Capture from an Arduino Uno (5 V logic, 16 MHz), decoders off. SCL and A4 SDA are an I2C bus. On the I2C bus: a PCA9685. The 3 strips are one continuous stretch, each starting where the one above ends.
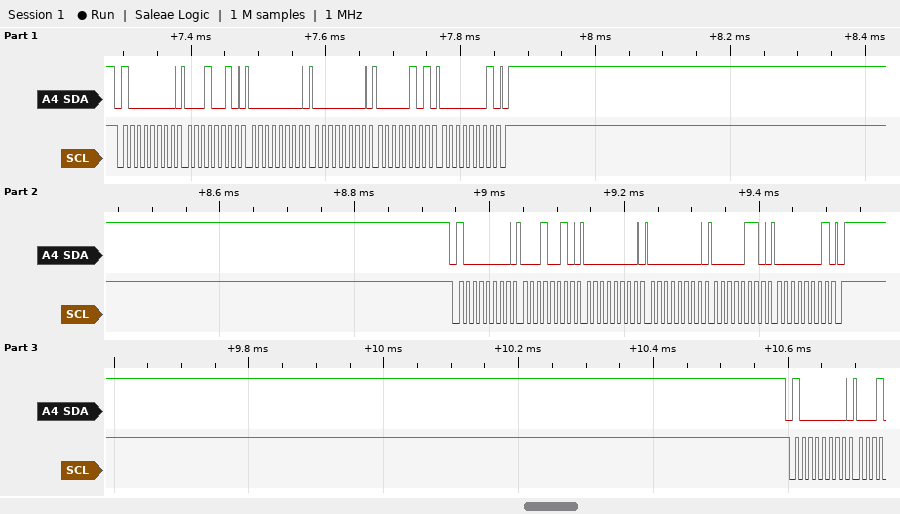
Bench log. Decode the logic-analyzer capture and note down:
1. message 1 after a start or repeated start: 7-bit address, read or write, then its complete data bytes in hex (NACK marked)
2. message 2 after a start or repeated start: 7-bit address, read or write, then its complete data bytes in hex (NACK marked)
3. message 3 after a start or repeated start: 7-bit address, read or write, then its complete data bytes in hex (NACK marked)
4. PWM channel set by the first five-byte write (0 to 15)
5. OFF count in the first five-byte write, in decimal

0x40 write: 12 00 00 05 01
0x40 write: 12 00 00 06 01
0x40 write
3
261
